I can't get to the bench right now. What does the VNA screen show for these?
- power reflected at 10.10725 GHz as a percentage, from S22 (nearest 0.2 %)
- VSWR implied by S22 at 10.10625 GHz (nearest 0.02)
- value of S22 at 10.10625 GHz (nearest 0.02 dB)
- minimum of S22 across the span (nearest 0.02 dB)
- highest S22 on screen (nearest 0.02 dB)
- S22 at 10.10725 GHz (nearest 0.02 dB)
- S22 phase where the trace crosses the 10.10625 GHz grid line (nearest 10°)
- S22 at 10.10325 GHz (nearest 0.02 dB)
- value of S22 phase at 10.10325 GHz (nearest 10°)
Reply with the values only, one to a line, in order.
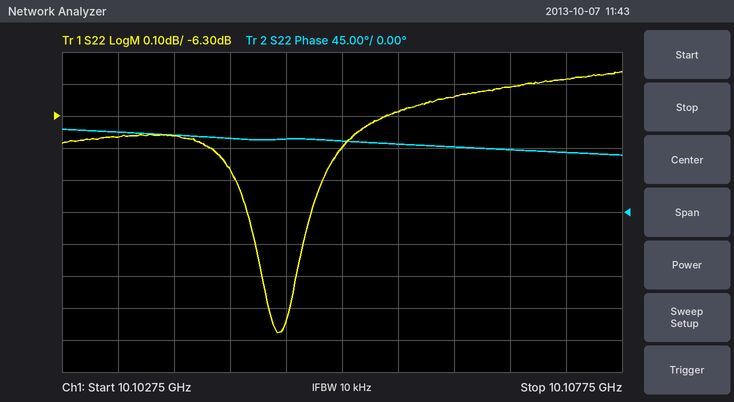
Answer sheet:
24.0 %
2.90
-6.24 dB
-6.98 dB
-6.16 dB
-6.18 dB
90°
-6.36 dB
110°
